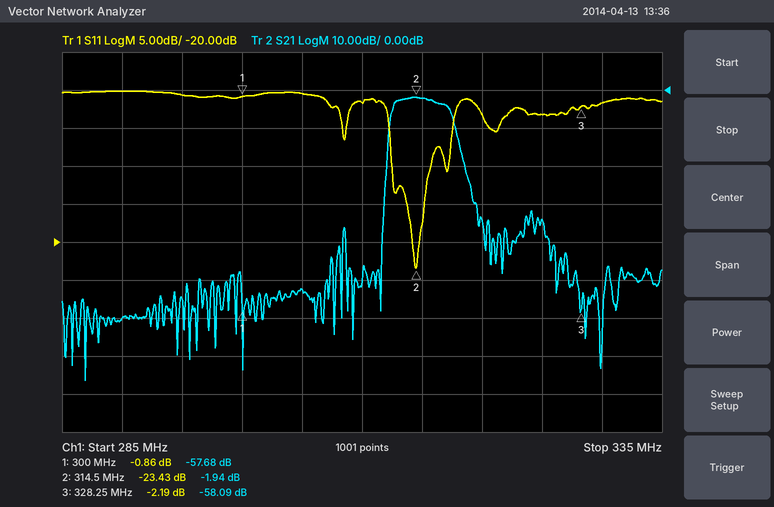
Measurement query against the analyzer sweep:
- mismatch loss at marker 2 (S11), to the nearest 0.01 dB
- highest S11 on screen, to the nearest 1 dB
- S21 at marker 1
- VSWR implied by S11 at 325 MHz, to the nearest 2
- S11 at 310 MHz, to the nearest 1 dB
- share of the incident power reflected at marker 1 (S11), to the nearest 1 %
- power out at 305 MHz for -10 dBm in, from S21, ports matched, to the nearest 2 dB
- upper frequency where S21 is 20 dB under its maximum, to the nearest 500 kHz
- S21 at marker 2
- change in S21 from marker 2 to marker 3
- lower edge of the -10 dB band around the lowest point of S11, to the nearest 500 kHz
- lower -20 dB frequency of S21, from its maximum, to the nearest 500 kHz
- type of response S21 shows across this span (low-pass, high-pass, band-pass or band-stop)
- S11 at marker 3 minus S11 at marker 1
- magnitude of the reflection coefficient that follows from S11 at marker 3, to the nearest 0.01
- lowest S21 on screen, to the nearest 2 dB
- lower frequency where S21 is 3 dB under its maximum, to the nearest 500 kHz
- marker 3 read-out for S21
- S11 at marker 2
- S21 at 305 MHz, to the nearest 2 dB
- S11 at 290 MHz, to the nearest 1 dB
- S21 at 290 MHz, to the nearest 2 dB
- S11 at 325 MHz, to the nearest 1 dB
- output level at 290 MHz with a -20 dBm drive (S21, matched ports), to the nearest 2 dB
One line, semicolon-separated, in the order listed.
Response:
0.02 dB; 0 dB; -57.68 dB; 6; -2 dB; 82 %; -62 dBm; 318.5 MHz; -1.94 dB; -56.15 dB; 312.5 MHz; 312.0 MHz; band-pass; -1.33 dB; 0.78; -76 dB; 312.5 MHz; -58.09 dB; -23.43 dB; -52 dB; 0 dB; -60 dB; -3 dB; -80 dBm
